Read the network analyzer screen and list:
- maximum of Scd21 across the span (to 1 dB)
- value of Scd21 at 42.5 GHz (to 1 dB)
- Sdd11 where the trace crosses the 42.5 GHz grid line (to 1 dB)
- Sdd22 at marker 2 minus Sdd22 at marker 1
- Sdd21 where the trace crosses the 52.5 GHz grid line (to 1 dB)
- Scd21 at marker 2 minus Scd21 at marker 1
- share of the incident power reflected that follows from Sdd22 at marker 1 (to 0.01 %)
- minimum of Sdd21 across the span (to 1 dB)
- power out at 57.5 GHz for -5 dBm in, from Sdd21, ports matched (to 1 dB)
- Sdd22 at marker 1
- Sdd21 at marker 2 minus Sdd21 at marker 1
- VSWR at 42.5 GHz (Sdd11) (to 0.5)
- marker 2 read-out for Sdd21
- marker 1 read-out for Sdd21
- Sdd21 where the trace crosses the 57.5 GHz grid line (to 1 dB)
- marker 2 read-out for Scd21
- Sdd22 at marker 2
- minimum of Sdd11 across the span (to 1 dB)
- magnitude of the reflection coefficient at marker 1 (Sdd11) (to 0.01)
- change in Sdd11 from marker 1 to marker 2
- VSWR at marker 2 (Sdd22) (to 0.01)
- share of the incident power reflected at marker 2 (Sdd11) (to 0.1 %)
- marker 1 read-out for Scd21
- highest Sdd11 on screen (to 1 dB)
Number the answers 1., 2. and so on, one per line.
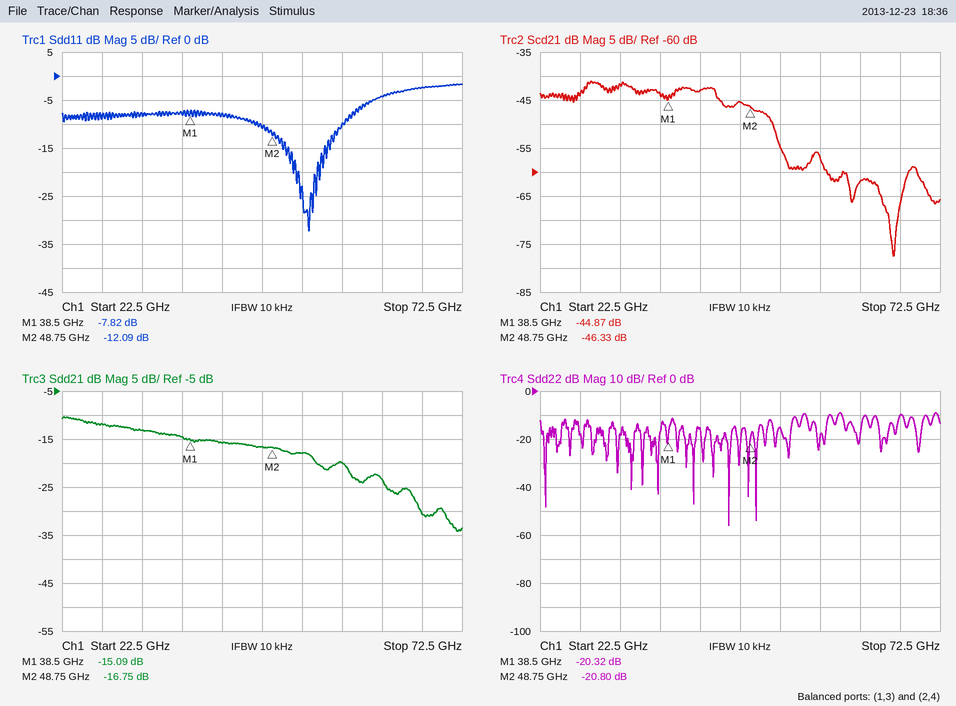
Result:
1. -41 dB
2. -43 dB
3. -8 dB
4. -0.48 dB
5. -18 dB
6. -1.46 dB
7. 0.93 %
8. -34 dB
9. -25 dBm
10. -20.32 dB
11. -1.66 dB
12. 2.5
13. -16.75 dB
14. -15.09 dB
15. -20 dB
16. -46.33 dB
17. -20.80 dB
18. -32 dB
19. 0.41
20. -4.27 dB
21. 1.20
22. 6.2 %
23. -44.87 dB
24. -2 dB
